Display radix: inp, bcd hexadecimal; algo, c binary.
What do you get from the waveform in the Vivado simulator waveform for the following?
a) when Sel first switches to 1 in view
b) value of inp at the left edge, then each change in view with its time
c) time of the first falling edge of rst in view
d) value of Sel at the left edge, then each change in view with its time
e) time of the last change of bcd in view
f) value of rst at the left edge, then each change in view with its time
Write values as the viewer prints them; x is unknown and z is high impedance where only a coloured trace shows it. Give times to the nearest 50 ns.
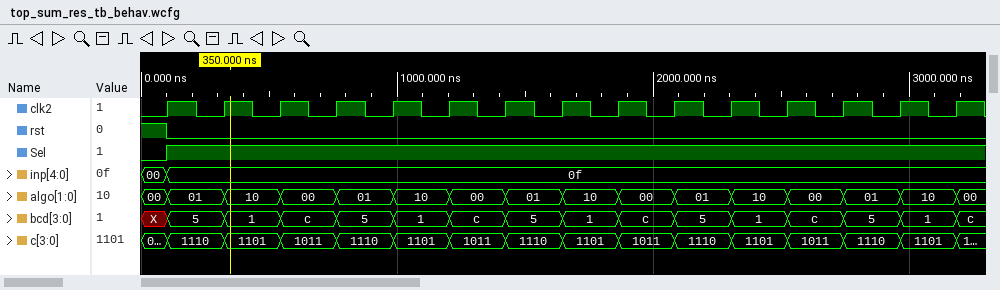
100 ns
00, 0f at 100 ns
100 ns
0, 1 at 100 ns
3200 ns
1, 0 at 100 ns
